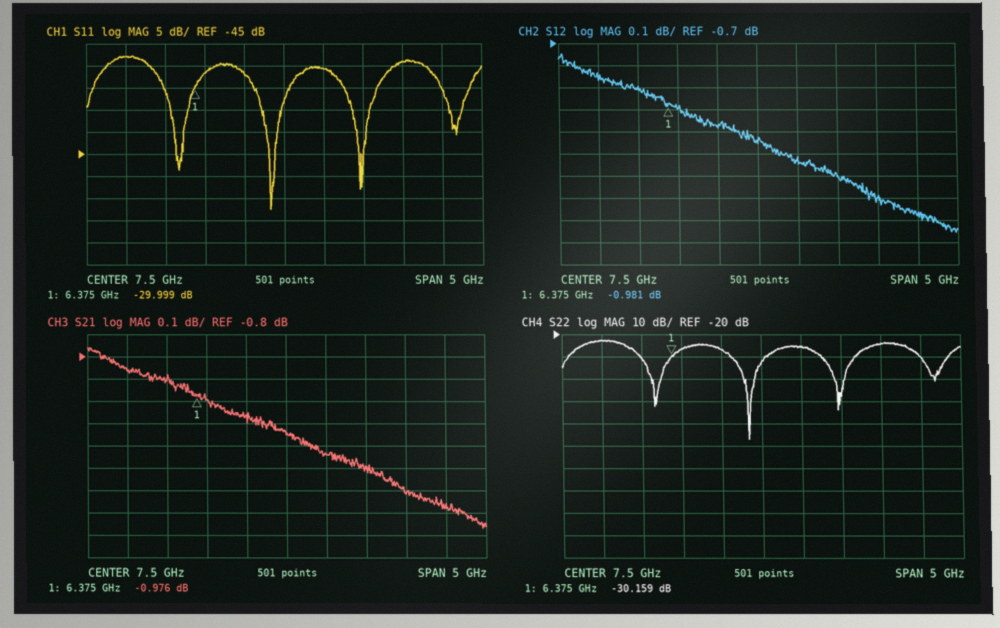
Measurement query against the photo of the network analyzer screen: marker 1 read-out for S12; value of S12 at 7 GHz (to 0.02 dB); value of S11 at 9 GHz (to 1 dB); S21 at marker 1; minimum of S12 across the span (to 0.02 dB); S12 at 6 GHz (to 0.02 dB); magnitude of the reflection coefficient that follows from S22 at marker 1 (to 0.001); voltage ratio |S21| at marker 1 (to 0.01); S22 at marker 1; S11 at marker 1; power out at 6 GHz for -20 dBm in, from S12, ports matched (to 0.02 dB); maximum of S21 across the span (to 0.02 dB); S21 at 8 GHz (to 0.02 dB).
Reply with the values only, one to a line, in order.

-0.981 dB
-1.08 dB
-24 dB
-0.976 dB
-1.56 dB
-0.90 dB
0.031
0.89
-30.159 dB
-29.999 dB
-20.90 dBm
-0.76 dB
-1.24 dB
